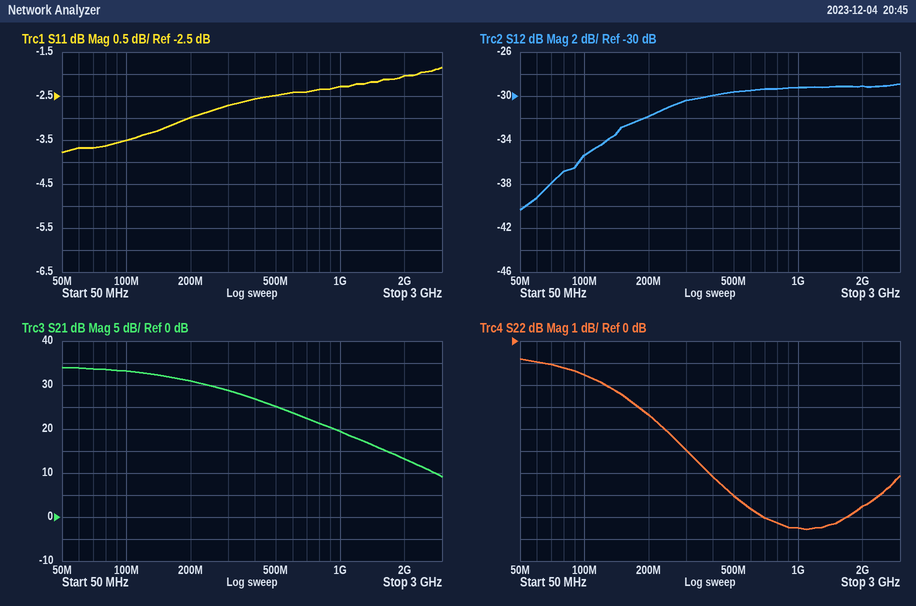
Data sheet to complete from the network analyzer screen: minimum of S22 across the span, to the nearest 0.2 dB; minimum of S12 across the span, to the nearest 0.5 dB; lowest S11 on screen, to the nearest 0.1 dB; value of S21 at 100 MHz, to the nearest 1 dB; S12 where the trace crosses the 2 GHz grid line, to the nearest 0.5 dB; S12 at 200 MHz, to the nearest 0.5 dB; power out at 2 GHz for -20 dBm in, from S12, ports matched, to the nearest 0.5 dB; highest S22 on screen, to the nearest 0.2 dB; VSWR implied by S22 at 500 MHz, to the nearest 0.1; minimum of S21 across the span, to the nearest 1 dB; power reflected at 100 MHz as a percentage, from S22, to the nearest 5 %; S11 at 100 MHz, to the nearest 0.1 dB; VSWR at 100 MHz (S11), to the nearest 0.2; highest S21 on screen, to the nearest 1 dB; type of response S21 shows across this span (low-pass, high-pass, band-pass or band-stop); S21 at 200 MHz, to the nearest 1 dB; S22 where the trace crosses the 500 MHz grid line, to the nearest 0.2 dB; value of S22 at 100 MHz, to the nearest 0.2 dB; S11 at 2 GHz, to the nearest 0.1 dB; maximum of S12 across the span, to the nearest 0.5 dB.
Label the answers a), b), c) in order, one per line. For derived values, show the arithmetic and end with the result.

a) -8.6 dB
b) -40.5 dB
c) -3.8 dB
d) 33 dB
e) -29.0 dB
f) -32.0 dB
g) -20 dBm + (-29.0 dB) = -49.0 dBm
h) -0.8 dB
i) |Γ| = 10^(-7/20) = 0.4467; VSWR = (1 + 0.4467)/(1 − 0.4467) ≈ 2.6
j) 9 dB
k) 10^(-1.6/10) ≈ 69.2 %, so 70 % to the nearest 5 %
l) -3.5 dB
m) |Γ| = 10^(-3.5/20) = 0.6683; VSWR = (1 + 0.6683)/(1 − 0.6683) ≈ 5.0
n) 34 dB
o) low-pass
p) 31 dB
q) -7.0 dB
r) -1.6 dB
s) -2.0 dB
t) -29.0 dB
